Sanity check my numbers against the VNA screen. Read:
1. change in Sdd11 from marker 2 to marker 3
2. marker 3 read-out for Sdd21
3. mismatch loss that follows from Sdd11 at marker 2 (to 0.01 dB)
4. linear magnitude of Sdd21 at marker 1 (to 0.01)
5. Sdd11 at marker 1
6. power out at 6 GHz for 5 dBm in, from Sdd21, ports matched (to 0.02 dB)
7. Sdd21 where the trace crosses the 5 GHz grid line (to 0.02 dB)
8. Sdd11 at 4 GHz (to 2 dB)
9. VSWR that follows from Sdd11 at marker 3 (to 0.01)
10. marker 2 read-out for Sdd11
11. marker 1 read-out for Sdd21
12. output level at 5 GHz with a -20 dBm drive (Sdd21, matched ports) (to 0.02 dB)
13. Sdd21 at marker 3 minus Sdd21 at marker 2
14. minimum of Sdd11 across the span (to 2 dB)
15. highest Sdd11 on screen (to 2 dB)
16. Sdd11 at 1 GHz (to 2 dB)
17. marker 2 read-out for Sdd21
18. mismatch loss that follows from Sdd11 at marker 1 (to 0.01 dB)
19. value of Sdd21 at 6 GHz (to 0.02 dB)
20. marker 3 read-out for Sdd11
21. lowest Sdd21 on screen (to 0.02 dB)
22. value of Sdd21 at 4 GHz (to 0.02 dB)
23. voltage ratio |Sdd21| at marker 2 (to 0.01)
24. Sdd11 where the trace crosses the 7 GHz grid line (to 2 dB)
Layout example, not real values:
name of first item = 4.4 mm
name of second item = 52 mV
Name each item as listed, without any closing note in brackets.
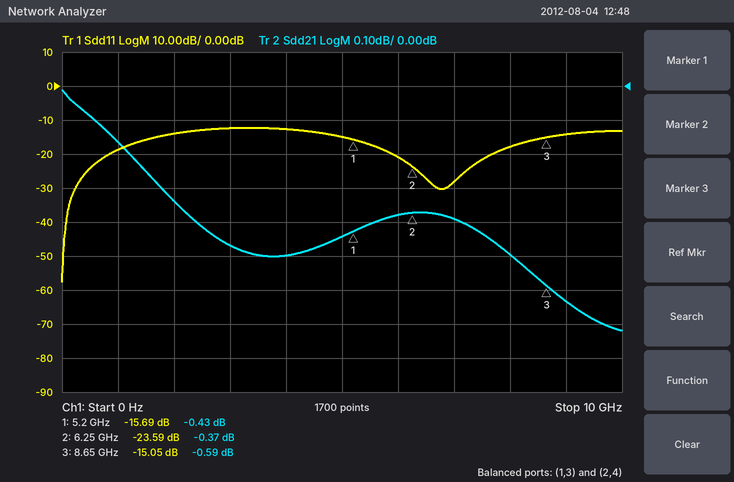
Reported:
change in Sdd11 from marker 2 to marker 3 = 8.54 dB
marker 3 read-out for Sdd21 = -0.59 dB
mismatch loss that follows from Sdd11 at marker 2 = 0.02 dB
linear magnitude of Sdd21 at marker 1 = 0.95
Sdd11 at marker 1 = -15.69 dB
power out at 6 GHz for 5 dBm in, from Sdd21, ports matched = 4.62 dBm
Sdd21 where the trace crosses the 5 GHz grid line = -0.44 dB
Sdd11 at 4 GHz = -12 dB
VSWR that follows from Sdd11 at marker 3 = 1.43
marker 2 read-out for Sdd11 = -23.59 dB
marker 1 read-out for Sdd21 = -0.43 dB
output level at 5 GHz with a -20 dBm drive (Sdd21, matched ports) = -20.44 dBm
Sdd21 at marker 3 minus Sdd21 at marker 2 = -0.22 dB
minimum of Sdd11 across the span = -58 dB
highest Sdd11 on screen = -12 dB
Sdd11 at 1 GHz = -18 dB
marker 2 read-out for Sdd21 = -0.37 dB
mismatch loss that follows from Sdd11 at marker 1 = 0.12 dB
value of Sdd21 at 6 GHz = -0.38 dB
marker 3 read-out for Sdd11 = -15.05 dB
lowest Sdd21 on screen = -0.72 dB
value of Sdd21 at 4 GHz = -0.50 dB
voltage ratio |Sdd21| at marker 2 = 0.96
Sdd11 where the trace crosses the 7 GHz grid line = -28 dB
